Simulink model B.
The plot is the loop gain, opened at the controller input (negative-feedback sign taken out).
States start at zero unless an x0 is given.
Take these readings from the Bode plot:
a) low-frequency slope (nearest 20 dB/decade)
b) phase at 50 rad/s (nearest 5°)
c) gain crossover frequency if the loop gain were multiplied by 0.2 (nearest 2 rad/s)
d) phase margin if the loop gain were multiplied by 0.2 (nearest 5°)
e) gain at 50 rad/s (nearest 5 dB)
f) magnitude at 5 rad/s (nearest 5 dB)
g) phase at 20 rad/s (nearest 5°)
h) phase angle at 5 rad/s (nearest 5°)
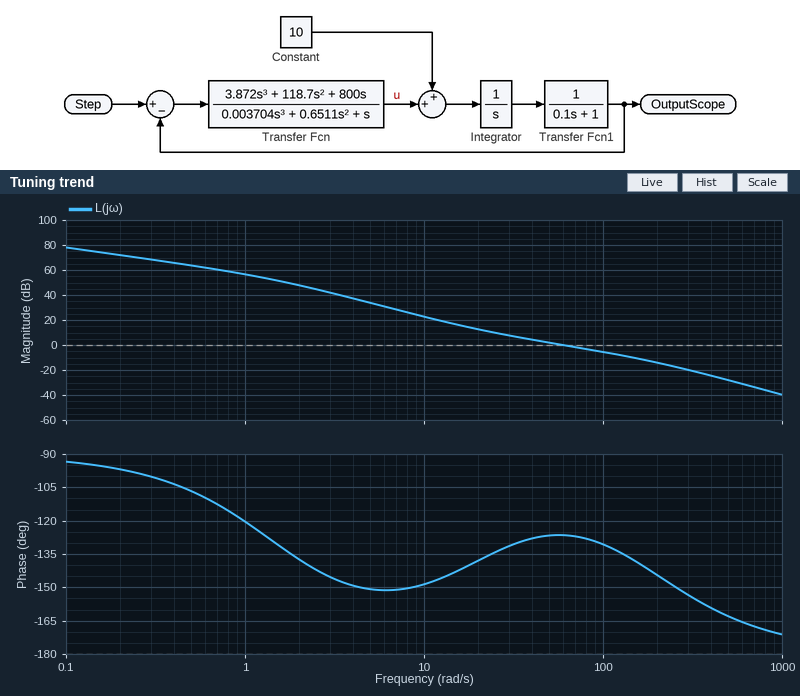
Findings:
-20 dB/decade
-125°
18 rad/s
40°
0 dB
35 dB
-140°
-150°
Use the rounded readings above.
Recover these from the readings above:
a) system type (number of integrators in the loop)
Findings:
1
